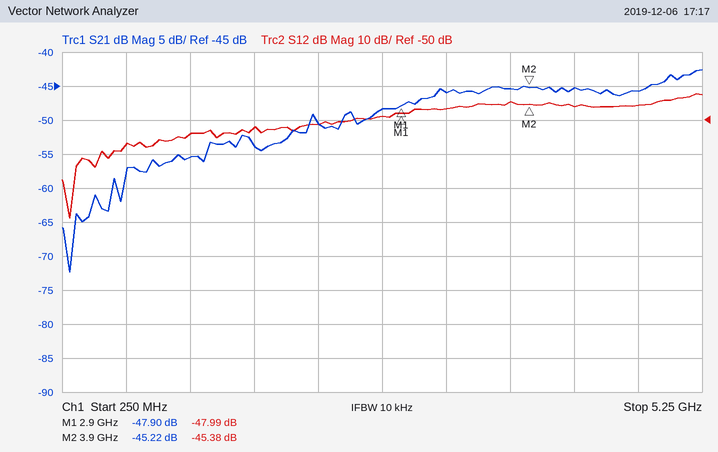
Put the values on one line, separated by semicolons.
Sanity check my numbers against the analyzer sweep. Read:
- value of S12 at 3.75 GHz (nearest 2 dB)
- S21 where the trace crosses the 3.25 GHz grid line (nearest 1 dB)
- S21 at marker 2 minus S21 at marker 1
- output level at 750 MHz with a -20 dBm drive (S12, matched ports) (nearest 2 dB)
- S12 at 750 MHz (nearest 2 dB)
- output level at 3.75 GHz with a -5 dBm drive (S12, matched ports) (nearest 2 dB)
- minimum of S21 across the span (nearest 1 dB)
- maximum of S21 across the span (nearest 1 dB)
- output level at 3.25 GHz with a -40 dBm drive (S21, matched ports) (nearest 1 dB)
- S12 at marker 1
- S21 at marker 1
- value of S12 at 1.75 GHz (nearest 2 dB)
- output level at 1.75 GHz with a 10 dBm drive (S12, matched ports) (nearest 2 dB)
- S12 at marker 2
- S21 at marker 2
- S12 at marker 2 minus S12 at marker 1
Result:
-44 dB; -46 dB; 2.68 dB; -78 dBm; -58 dB; -50 dBm; -72 dB; -43 dB; -86 dBm; -47.99 dB; -47.90 dB; -52 dB; -42 dBm; -45.38 dB; -45.22 dB; 2.61 dB
